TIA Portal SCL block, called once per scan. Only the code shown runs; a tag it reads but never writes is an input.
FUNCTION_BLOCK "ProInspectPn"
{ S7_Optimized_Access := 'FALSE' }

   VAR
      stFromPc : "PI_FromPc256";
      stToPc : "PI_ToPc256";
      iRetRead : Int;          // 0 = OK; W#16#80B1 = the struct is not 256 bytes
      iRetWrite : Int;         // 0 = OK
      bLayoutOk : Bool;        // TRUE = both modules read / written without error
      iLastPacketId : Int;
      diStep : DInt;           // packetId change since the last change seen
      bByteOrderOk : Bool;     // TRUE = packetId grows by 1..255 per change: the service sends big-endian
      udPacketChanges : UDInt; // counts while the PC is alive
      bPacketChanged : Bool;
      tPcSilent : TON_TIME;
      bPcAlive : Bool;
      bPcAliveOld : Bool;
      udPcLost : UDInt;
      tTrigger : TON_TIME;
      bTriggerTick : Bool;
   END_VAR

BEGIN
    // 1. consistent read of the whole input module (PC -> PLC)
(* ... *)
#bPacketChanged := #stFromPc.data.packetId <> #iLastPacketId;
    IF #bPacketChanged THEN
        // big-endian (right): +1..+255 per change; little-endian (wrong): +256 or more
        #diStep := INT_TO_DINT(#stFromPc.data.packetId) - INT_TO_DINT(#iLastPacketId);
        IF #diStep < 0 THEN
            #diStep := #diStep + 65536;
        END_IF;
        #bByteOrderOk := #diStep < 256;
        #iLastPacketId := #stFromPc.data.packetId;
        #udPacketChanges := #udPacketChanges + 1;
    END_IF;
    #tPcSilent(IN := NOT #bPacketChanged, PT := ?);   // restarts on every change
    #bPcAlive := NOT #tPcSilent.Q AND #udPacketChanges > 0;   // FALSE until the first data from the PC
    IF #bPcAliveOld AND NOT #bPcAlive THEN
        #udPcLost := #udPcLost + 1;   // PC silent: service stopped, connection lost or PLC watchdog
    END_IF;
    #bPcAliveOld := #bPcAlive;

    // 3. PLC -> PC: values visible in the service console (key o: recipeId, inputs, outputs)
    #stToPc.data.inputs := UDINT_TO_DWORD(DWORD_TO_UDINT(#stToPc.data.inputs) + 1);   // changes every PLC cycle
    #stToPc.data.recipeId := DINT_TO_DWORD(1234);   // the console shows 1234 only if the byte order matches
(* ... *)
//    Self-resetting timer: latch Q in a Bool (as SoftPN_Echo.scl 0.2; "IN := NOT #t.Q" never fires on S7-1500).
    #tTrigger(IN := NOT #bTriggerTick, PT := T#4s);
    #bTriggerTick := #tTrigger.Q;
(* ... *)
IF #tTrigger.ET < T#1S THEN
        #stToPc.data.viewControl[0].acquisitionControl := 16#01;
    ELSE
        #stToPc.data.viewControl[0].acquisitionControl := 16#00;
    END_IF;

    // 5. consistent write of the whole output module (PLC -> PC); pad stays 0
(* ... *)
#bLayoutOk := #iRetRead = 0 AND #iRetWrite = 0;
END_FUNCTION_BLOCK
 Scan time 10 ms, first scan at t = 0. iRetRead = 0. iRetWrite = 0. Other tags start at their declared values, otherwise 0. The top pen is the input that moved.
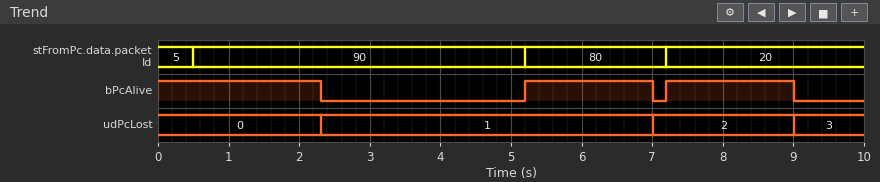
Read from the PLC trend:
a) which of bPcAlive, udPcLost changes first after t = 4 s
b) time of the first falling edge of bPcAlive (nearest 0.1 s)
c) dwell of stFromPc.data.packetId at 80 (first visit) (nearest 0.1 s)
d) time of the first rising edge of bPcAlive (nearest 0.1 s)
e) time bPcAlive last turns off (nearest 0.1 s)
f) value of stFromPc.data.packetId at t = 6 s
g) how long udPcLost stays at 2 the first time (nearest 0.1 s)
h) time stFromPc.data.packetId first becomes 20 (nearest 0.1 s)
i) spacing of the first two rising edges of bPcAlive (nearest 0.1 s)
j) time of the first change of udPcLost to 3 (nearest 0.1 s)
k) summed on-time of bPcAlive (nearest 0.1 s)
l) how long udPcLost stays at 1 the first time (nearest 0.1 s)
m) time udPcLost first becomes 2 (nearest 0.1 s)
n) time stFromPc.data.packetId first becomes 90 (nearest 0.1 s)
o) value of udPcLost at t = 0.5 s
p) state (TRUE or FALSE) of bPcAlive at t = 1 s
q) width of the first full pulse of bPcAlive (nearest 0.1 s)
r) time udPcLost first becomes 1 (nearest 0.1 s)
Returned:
bPcAlive
2.3 s
2.0 s
5.2 s
9.0 s
80
2.0 s
7.2 s
2.0 s
9.0 s
5.9 s
4.7 s
7.0 s
0.5 s
0
TRUE
1.8 s
2.3 s
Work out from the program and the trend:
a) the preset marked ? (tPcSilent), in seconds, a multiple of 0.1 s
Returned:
1.8 s
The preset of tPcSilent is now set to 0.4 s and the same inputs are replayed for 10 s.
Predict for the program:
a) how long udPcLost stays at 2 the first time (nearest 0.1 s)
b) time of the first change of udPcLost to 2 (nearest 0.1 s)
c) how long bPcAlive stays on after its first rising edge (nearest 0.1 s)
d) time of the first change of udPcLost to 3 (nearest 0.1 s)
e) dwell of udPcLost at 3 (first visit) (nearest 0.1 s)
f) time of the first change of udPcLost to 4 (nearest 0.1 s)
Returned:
4.7 s
0.9 s
0.4 s
5.6 s
2.0 s
7.6 s
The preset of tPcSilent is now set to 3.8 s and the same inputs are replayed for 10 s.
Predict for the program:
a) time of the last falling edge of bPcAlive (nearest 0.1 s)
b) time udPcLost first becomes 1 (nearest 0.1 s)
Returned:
4.3 s
4.3 s
